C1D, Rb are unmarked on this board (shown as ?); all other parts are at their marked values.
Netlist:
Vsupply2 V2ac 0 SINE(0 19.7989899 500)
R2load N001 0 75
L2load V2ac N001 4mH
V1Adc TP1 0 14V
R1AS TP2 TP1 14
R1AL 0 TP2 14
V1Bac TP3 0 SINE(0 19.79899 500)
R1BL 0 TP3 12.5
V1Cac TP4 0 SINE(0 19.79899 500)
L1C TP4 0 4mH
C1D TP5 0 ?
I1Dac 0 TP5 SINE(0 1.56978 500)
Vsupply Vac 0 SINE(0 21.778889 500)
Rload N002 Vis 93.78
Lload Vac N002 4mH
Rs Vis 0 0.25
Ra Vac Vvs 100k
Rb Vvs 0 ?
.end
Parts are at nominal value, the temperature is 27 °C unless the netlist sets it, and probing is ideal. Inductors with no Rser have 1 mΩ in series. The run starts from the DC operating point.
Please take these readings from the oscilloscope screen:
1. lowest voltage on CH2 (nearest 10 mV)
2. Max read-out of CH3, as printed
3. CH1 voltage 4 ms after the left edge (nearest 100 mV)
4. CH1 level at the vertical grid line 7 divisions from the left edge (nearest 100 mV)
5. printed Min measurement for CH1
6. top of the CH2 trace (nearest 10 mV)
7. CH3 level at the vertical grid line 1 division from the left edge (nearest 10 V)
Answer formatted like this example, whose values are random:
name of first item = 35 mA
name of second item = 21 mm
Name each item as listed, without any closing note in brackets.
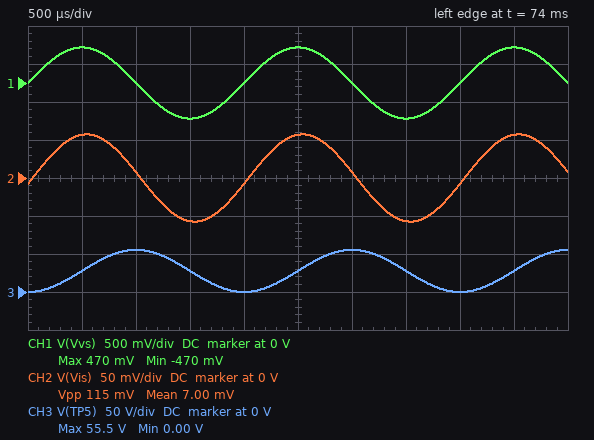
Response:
lowest voltage on CH2 = -60 mV
Max read-out of CH3, as printed = 55.5 V
CH1 voltage 4 ms after the left edge = 0 V
CH1 level at the vertical grid line 7 divisions from the left edge = -500 mV
printed Min measurement for CH1 = -470 mV
top of the CH2 trace = 60 mV
CH3 level at the vertical grid line 1 division from the left edge = 30 V
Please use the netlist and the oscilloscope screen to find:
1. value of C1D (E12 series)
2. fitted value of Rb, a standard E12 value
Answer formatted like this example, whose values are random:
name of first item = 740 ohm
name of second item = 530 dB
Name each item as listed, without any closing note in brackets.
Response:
value of C1D = 18 µF
fitted value of Rb, a standard E12 value = 2.2 kΩ
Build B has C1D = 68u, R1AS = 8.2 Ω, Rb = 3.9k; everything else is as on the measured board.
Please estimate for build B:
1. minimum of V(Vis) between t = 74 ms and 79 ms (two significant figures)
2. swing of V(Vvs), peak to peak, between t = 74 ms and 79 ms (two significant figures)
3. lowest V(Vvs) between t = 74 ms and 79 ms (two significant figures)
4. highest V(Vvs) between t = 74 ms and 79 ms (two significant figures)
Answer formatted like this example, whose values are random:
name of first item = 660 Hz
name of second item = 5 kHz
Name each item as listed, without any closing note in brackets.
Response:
minimum of V(Vis) between t = 74 ms and 79 ms = -57 mV
swing of V(Vvs), peak to peak, between t = 74 ms and 79 ms = 1.6 V
lowest V(Vvs) between t = 74 ms and 79 ms = -820 mV
highest V(Vvs) between t = 74 ms and 79 ms = 820 mV
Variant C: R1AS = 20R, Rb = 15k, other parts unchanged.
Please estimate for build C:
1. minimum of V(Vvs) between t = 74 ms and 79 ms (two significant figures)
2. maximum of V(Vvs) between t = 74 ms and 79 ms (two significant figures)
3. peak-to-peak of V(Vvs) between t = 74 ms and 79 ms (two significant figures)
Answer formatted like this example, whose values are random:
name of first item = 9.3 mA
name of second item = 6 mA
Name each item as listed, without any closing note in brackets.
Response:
minimum of V(Vvs) between t = 74 ms and 79 ms = -2.8 V
maximum of V(Vvs) between t = 74 ms and 79 ms = 2.8 V
peak-to-peak of V(Vvs) between t = 74 ms and 79 ms = 5.7 V
